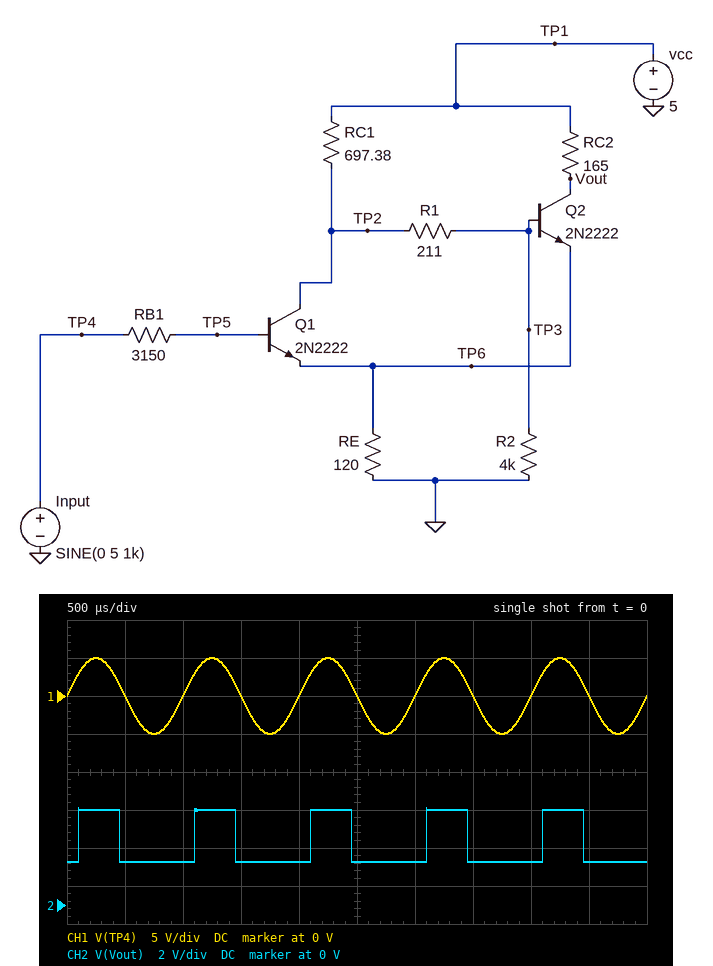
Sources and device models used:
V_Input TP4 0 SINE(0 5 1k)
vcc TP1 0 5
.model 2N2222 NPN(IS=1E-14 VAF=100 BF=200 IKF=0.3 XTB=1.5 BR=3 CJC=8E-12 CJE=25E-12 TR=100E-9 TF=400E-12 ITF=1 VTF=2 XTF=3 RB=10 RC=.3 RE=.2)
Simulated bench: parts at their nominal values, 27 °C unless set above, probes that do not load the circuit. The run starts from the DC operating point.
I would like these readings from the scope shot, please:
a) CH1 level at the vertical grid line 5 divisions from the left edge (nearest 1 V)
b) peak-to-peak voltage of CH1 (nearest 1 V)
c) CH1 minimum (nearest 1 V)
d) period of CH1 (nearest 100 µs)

0 V
10 V
-5 V
1.0 ms
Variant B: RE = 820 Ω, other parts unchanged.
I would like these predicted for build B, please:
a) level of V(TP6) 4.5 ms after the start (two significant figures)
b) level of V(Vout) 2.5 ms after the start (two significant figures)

3.4 V
4.3 V
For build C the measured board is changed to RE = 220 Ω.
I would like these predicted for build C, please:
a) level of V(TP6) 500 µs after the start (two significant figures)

2.9 V
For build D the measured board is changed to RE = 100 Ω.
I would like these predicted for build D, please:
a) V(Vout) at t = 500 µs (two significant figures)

2.0 V
